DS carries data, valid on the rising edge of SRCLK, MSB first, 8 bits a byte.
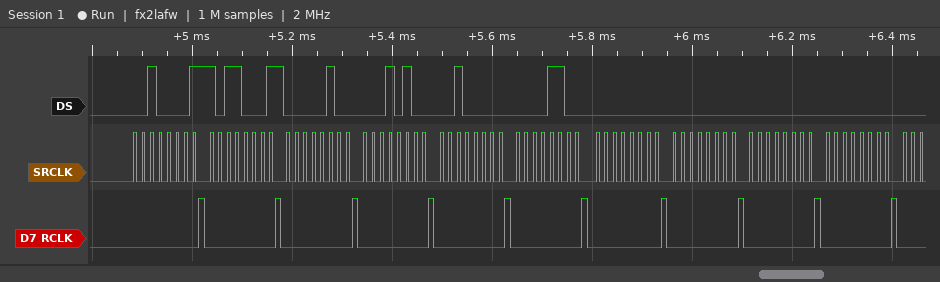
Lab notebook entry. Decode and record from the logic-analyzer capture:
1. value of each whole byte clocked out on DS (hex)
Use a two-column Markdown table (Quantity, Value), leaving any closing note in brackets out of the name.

| Quantity | Value |
|---|---|
| value of each whole byte clocked out on DS | 0x21 0xB1 0x04 0x14 0x20 0x0C 0x00 0x00 0x00 0x00 |
